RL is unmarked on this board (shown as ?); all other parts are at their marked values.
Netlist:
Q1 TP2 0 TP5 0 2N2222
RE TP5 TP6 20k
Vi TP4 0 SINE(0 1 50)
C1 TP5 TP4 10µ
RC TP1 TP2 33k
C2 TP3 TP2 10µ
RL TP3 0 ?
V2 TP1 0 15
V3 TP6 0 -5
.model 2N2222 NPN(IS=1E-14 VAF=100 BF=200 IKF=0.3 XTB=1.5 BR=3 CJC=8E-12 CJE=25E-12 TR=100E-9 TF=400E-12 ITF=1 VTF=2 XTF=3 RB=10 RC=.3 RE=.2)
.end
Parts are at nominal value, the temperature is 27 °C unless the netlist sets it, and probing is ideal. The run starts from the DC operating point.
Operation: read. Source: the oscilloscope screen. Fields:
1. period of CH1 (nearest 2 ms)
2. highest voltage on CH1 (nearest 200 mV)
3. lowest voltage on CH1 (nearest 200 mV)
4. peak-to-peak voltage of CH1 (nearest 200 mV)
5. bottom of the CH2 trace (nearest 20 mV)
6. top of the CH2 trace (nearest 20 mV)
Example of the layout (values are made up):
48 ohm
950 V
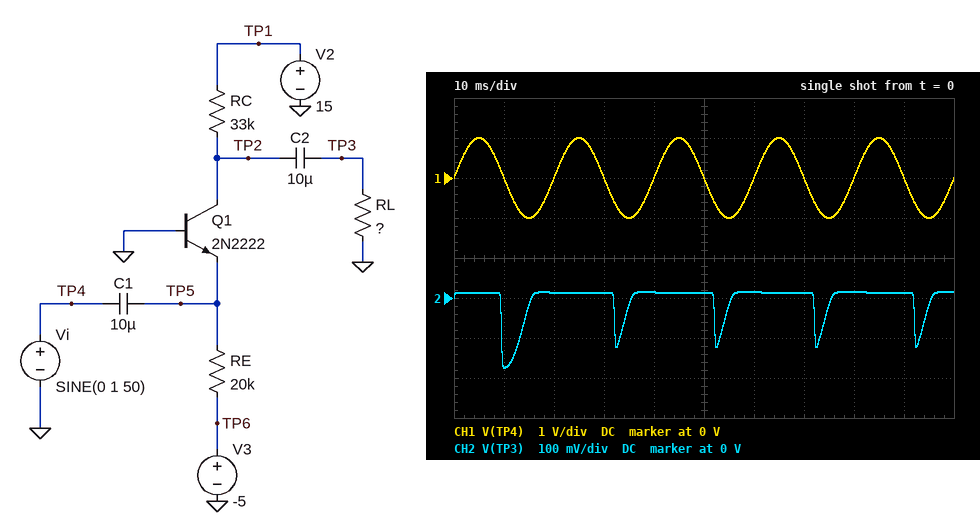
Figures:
20 ms
1.0 V
-1.0 V
2.0 V
-180 mV
20 mV
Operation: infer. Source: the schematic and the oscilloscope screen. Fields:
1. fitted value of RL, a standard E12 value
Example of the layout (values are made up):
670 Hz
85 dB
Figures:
56 Ω
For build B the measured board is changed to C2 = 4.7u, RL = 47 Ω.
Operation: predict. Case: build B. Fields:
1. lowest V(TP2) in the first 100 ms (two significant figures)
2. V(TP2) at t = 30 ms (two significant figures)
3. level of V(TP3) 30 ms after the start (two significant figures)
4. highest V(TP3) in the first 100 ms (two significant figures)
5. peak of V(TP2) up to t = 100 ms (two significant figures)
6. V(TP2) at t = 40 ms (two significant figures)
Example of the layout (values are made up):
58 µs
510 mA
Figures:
5.7 V
6.5 V
12 mV
13 mV
8.2 V
6.0 V
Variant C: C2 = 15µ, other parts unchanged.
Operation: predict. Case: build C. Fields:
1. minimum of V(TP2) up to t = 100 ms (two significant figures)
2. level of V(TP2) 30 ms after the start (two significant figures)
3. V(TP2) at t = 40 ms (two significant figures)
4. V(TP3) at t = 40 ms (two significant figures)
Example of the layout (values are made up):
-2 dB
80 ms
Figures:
7.0 V
7.4 V
7.2 V
13 mV
